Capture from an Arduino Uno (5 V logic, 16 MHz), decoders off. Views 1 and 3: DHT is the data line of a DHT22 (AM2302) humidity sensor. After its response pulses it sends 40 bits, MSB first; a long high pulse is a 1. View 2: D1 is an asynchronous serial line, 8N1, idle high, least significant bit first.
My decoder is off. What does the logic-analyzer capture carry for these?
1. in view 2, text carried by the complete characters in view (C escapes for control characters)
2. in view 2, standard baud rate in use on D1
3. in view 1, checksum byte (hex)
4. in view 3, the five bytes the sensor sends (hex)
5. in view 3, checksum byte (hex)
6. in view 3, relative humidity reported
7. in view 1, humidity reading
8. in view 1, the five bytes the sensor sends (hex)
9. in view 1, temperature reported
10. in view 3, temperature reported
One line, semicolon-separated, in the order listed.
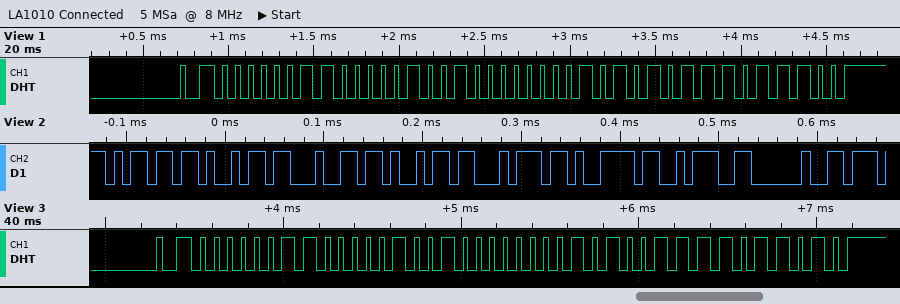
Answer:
"midity: "; 115200 baud; 0xDC; 03 04 80 53 DA; 0xDA; 77.2 %; 77.2 %; 03 04 80 55 DC; -8.5 °C; -8.3 °C
